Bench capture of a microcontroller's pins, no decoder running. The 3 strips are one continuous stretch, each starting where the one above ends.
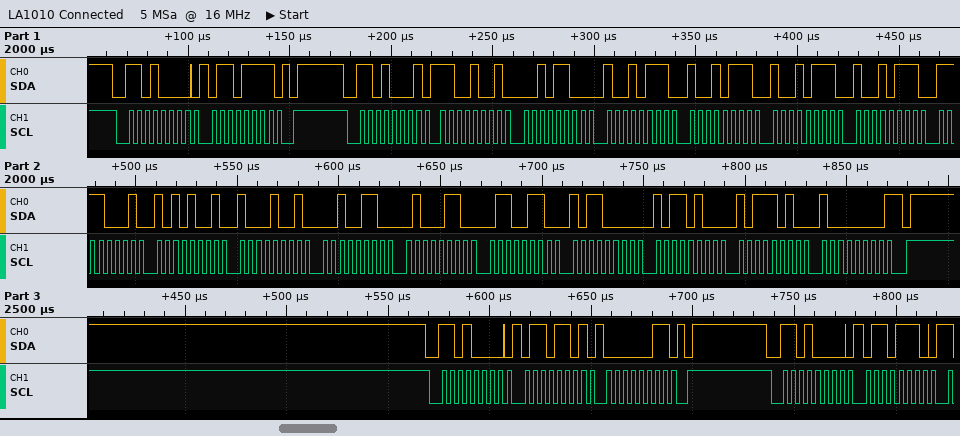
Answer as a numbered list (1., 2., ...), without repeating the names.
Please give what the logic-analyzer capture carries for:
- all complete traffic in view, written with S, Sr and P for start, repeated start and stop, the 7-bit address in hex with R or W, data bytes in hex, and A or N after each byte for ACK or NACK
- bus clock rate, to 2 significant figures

1. S 68W A 6F A P S 68R A C9 A 2C A 97 A 97 A 97 A 97 A F1 A A9 A 89 A 26 A 46 A 66 A B0 A B4 A BA A 80 N P S 68W A 6D A 03 A P S 68W A 6E A
2. 250 kHz
